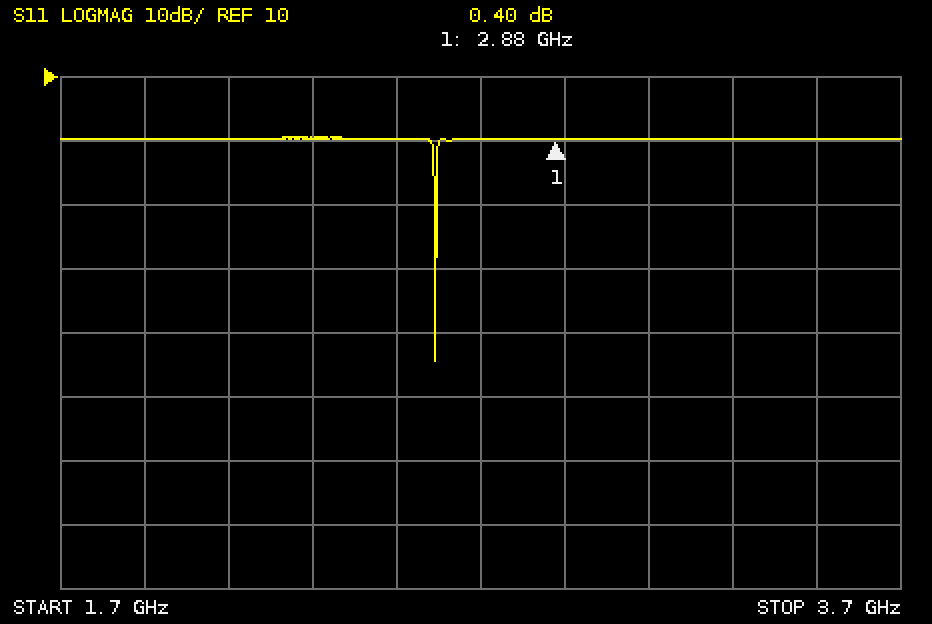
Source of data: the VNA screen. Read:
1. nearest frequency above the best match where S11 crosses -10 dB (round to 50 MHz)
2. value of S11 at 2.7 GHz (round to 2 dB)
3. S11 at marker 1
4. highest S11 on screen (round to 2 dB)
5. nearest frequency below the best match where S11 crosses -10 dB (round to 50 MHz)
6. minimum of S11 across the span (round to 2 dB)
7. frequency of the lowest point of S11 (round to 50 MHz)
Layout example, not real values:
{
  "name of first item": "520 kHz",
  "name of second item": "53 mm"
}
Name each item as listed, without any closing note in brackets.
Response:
{
  "nearest frequency above the best match where S11 crosses -10 dB": "2.60 GHz",
  "value of S11 at 2.7 GHz": "0 dB",
  "S11 at marker 1": "0.40 dB",
  "highest S11 on screen": "0 dB",
  "nearest frequency below the best match where S11 crosses -10 dB": "2.60 GHz",
  "minimum of S11 across the span": "-34 dB",
  "frequency of the lowest point of S11": "2.60 GHz"
}
